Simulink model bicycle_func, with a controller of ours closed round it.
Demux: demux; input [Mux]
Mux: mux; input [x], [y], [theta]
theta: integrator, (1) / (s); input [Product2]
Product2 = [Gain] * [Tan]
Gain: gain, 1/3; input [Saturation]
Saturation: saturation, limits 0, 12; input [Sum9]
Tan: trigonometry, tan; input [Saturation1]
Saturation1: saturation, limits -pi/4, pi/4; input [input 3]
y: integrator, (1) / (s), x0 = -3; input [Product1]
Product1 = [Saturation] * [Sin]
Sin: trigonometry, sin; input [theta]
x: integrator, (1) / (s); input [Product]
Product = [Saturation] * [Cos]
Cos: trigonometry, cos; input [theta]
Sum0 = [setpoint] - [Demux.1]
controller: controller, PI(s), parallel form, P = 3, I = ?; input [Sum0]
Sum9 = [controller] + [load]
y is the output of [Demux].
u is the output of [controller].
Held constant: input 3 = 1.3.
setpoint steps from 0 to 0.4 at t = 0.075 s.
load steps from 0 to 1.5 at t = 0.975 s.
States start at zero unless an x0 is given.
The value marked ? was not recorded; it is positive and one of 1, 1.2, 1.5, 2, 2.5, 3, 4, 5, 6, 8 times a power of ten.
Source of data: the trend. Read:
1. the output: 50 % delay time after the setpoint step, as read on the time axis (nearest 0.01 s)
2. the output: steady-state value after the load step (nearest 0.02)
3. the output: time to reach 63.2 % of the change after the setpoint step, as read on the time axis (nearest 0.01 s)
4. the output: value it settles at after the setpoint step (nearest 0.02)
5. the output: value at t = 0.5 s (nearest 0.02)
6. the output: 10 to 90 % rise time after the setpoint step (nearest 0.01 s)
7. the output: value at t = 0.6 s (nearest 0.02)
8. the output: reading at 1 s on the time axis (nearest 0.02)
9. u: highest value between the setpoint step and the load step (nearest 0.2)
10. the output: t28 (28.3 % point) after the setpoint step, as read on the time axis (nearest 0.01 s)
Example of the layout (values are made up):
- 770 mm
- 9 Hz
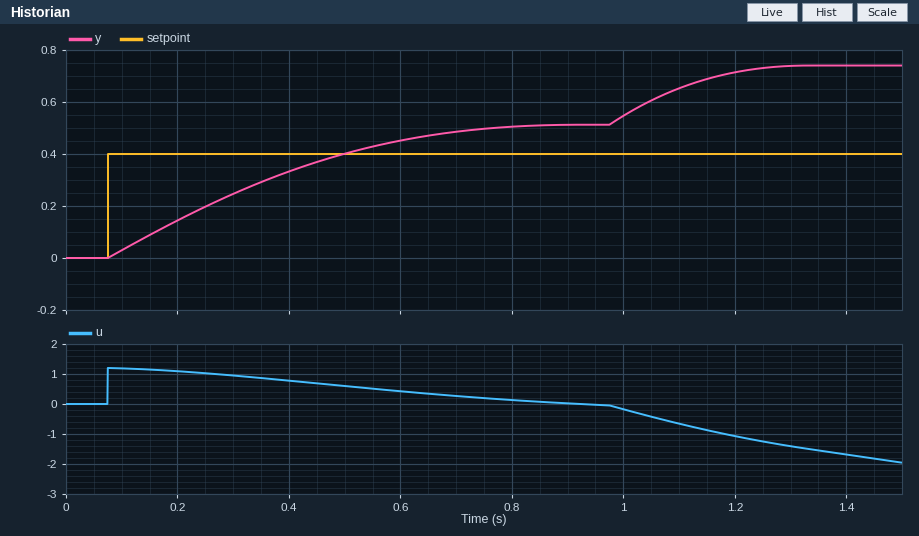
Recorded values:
- 0.31 s
- 0.74
- 0.39 s
- 0.52
- 0.40
- 0.51 s
- 0.46
- 0.54
- 1.2
- 0.20 s
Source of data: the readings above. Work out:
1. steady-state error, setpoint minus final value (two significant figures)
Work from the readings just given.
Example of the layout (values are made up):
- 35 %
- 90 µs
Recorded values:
- -0.12
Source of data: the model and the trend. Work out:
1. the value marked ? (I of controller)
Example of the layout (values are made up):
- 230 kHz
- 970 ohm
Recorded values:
- 8
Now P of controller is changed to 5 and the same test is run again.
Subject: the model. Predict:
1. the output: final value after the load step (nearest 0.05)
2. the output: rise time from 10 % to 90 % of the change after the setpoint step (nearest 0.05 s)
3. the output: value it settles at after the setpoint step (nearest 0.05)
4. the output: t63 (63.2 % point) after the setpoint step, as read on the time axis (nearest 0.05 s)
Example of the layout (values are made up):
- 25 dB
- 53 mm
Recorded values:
- 0.65
- 0.40 s
- 0.45
- 0.30 s
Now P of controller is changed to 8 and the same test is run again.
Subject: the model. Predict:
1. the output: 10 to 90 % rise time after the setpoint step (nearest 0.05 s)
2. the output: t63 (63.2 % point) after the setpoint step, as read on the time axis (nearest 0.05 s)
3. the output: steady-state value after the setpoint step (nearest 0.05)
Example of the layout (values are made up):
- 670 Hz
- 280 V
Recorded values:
- 0.25 s
- 0.20 s
- 0.45
